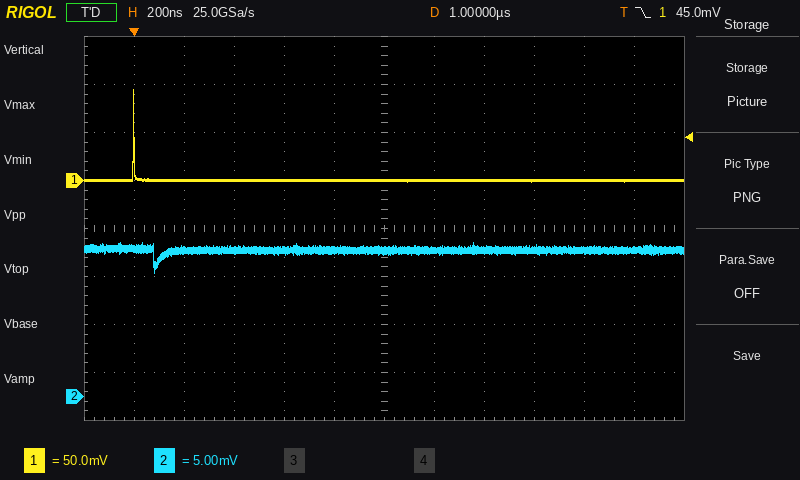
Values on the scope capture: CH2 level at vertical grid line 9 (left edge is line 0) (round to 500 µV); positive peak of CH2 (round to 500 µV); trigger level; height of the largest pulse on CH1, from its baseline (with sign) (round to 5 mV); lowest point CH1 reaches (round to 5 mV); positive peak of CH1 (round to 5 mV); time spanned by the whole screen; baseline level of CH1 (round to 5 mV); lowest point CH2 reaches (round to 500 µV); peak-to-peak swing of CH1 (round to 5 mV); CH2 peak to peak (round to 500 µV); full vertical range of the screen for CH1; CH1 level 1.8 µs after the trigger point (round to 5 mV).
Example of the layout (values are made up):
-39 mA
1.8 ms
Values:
15.5 mV
16.0 mV
45.0 mV
+95 mV
0 mV
95 mV
2.4 µs
0 mV
13.0 mV
95 mV
3.0 mV
400 mV
0 mV
